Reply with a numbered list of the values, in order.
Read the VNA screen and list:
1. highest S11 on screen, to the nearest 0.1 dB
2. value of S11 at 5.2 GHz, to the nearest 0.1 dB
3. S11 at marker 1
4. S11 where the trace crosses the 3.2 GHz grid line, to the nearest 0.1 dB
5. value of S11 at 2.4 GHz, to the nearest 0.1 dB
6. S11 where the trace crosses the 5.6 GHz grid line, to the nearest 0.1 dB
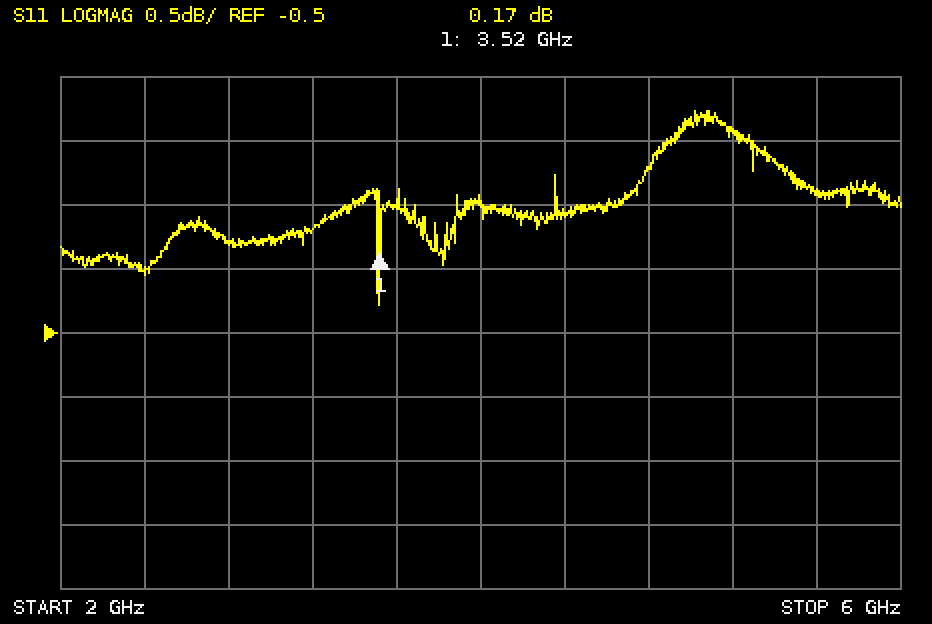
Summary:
1. 1.2 dB
2. 1.1 dB
3. 0.17 dB
4. 0.3 dB
5. 0.0 dB
6. 0.6 dB
